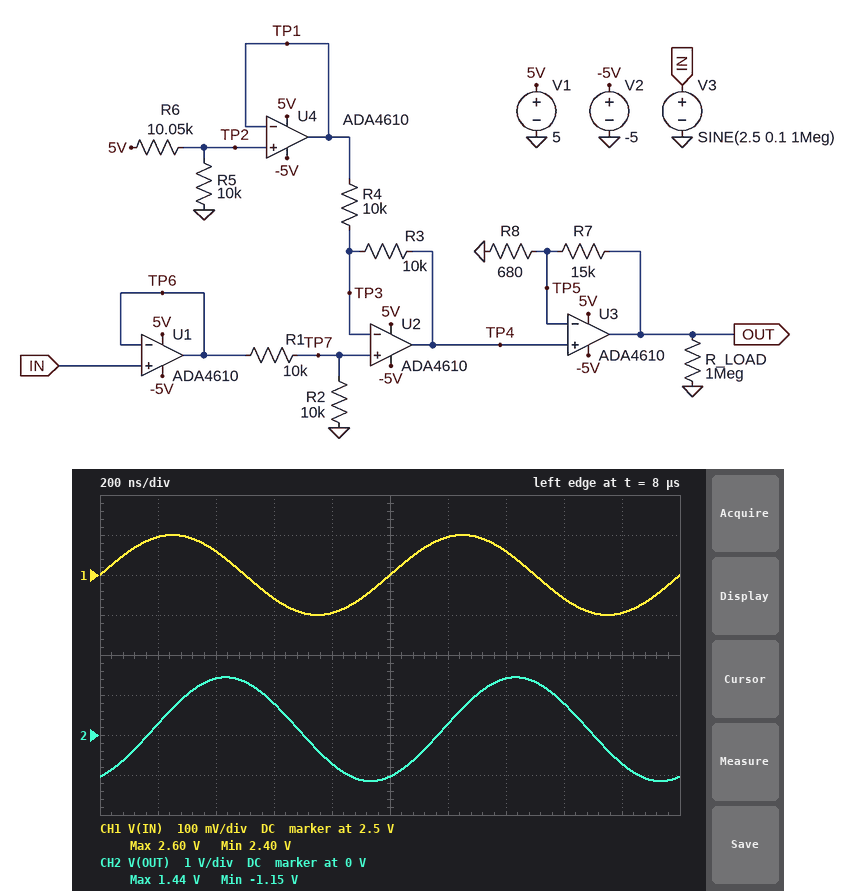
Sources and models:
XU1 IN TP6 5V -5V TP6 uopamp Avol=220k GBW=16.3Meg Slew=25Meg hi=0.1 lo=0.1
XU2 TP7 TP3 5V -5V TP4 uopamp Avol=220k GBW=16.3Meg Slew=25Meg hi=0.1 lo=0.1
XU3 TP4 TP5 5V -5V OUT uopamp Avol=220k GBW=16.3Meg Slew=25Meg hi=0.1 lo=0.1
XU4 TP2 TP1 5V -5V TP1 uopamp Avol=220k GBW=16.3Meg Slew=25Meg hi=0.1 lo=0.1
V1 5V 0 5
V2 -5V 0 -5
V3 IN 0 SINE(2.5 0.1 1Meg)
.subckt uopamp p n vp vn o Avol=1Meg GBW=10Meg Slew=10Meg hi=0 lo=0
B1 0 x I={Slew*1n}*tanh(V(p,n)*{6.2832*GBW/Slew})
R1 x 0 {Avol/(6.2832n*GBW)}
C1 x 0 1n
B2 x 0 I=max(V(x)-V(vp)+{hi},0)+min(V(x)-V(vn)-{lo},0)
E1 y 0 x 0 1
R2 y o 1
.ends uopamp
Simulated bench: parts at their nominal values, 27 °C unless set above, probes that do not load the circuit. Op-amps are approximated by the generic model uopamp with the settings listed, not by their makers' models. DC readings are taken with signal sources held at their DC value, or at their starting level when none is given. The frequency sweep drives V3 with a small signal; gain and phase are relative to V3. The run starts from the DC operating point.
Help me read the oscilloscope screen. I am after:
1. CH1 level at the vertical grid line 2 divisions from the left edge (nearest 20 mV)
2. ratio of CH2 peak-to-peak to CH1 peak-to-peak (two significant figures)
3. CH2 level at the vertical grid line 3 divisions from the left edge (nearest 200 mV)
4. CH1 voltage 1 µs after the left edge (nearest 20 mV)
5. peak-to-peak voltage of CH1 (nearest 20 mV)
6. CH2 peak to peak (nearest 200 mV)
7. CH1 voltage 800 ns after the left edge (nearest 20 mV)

2.56 V
13
800 mV
2.50 V
200 mV
2.6 V
2.40 V
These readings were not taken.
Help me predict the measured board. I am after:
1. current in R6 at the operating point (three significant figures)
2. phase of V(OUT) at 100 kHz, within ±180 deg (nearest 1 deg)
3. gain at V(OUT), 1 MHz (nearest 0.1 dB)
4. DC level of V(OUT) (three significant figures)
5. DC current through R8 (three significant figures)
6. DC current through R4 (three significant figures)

249 µA
-9 deg
22.4 dB
144 mV
9.17 µA
124 µA
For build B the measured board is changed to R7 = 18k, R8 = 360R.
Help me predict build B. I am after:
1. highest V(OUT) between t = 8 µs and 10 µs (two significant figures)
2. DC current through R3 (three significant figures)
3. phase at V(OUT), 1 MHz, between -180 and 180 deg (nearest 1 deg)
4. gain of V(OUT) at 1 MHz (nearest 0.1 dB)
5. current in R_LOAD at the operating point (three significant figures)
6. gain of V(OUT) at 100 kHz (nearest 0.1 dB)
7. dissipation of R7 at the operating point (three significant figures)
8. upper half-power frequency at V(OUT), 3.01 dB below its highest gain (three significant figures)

1.8 V
124 µA
-83 deg
23.7 dB
318 nA
33.7 dB
5.40 µW
319 kHz
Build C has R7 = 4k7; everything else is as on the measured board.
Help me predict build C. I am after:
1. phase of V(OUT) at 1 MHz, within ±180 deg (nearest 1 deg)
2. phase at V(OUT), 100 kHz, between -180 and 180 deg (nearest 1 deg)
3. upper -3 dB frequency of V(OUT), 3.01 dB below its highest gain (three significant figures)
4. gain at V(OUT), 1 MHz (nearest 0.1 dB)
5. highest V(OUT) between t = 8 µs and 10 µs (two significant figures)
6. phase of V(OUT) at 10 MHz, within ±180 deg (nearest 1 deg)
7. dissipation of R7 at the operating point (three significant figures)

-36 deg
-4 deg
1.92 MHz
17.0 dB
750 mV
-161 deg
395 nW
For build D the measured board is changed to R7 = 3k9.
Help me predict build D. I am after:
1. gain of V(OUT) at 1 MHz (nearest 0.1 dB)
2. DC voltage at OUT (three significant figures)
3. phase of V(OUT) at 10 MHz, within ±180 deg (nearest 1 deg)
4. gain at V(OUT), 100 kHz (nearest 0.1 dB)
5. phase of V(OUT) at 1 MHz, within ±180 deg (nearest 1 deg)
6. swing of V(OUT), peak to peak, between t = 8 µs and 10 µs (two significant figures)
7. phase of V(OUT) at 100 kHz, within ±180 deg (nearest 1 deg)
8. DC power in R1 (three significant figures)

15.8 dB
42.0 mV
-159 deg
16.6 dB
-33 deg
1.2 V
-3 deg
156 µW
